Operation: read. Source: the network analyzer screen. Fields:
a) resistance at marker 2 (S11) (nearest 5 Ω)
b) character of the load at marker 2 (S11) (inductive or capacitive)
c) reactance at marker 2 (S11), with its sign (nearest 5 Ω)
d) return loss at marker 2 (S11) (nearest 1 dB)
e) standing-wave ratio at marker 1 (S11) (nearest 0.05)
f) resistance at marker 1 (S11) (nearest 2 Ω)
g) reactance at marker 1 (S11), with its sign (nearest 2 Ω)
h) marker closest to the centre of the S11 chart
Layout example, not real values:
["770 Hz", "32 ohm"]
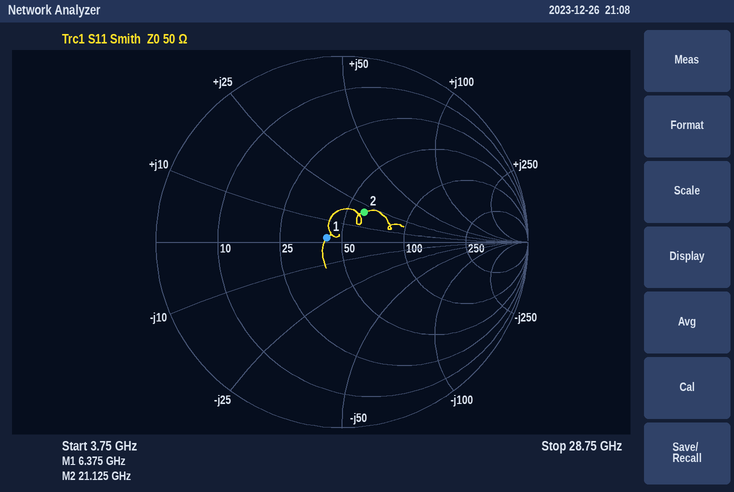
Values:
["60 Ω", "inductive", "+20 Ω", "14 dB", "1.20", "42 Ω", "+2 Ω", "marker 1"]
